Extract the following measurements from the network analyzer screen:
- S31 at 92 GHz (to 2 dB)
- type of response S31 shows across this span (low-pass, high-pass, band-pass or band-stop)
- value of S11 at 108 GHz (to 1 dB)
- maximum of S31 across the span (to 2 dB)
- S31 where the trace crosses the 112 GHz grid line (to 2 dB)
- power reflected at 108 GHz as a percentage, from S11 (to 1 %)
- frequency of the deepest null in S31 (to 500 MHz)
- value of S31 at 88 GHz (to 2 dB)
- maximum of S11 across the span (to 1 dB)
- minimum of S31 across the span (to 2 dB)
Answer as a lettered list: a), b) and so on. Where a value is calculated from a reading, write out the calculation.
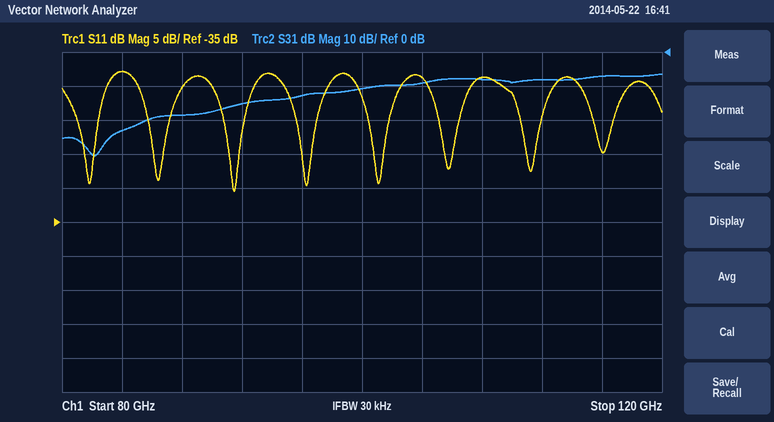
a) -16 dB
b) high-pass
c) -14 dB
d) -6 dB
e) -8 dB
f) 10^(-14/10) ≈ 4 %
g) 82.0 GHz
h) -18 dB
i) -13 dB
j) -30 dB
